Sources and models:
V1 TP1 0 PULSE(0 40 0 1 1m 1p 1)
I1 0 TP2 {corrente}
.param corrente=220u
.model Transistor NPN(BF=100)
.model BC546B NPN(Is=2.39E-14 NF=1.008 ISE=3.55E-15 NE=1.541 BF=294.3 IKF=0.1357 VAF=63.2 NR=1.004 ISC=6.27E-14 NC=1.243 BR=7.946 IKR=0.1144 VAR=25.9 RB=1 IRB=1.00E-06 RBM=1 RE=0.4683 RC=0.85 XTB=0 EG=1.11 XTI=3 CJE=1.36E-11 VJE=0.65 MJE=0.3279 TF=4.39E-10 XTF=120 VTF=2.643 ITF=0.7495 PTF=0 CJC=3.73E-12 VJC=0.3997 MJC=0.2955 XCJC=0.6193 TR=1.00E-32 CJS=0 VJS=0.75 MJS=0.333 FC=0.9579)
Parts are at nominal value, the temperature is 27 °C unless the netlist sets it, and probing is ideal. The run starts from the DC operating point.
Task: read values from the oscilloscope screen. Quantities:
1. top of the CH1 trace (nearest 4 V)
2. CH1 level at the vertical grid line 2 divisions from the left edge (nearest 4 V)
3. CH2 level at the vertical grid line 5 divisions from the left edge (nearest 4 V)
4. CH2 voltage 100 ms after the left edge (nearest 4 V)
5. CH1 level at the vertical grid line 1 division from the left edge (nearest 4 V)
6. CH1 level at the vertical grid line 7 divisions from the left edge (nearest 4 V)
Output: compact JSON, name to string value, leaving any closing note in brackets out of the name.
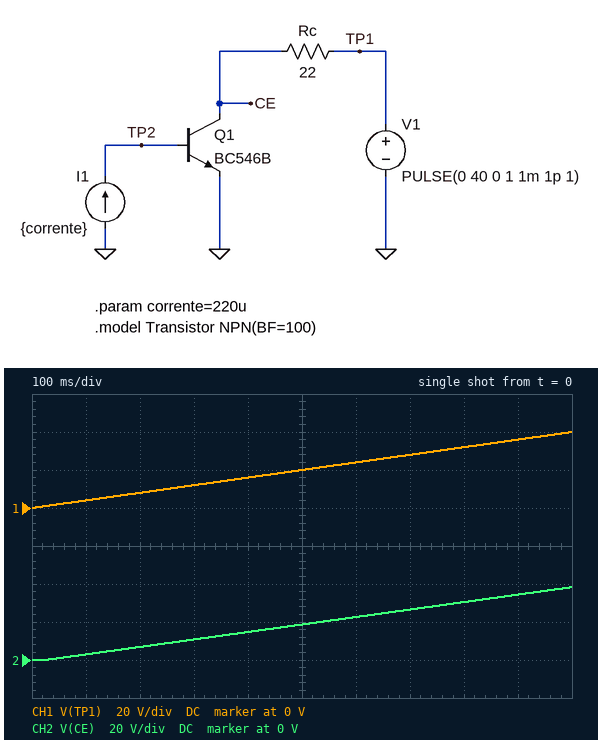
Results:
{"top of the CH1 trace": "40 V", "CH1 level at the vertical grid line 2 divisions from the left edge": "8 V", "CH2 level at the vertical grid line 5 divisions from the left edge": "20 V", "CH2 voltage 100 ms after the left edge": "4 V", "CH1 level at the vertical grid line 1 division from the left edge": "4 V", "CH1 level at the vertical grid line 7 divisions from the left edge": "28 V"}
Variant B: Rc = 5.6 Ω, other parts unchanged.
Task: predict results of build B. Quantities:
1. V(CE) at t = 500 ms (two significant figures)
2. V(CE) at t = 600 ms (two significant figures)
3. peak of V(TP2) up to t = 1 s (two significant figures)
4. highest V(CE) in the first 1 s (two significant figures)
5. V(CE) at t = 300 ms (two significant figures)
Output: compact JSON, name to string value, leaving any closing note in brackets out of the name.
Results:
{"V(CE) at t = 500 ms": "20 V", "V(CE) at t = 600 ms": "24 V", "peak of V(TP2) up to t = 1 s": "780 mV", "highest V(CE) in the first 1 s": "40 V", "V(CE) at t = 300 ms": "12 V"}
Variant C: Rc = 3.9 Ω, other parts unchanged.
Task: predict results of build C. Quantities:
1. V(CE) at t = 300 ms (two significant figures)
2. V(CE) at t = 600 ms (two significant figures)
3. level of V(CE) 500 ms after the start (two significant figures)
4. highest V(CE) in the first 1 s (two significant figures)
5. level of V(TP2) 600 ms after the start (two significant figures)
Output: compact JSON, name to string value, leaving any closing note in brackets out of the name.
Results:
{"V(CE) at t = 300 ms": "12 V", "V(CE) at t = 600 ms": "24 V", "level of V(CE) 500 ms after the start": "20 V", "highest V(CE) in the first 1 s": "40 V", "level of V(TP2) 600 ms after the start": "780 mV"}
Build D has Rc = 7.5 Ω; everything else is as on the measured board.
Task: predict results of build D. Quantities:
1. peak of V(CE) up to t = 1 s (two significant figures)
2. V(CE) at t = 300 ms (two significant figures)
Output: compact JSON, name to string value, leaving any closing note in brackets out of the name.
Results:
{"peak of V(CE) up to t = 1 s": "39 V", "V(CE) at t = 300 ms": "12 V"}
